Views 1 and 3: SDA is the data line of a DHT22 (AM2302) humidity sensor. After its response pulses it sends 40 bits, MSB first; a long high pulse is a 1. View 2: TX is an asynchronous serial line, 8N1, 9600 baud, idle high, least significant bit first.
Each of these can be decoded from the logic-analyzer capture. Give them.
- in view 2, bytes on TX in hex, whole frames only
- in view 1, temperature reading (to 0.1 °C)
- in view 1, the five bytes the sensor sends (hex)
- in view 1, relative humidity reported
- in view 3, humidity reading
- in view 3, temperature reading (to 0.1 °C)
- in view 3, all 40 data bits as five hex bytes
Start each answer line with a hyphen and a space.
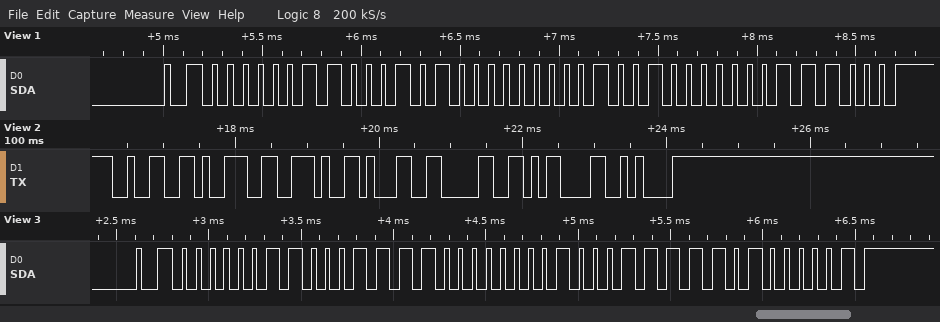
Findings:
- 0x32 0x39 0x2E 0x31 0x30 0x0D 0x0A
- 28.8 °C
- 03 14 01 20 38
- 78.8 %
- 79.8 %
- 28.7 °C
- 03 1E 01 1F 41
